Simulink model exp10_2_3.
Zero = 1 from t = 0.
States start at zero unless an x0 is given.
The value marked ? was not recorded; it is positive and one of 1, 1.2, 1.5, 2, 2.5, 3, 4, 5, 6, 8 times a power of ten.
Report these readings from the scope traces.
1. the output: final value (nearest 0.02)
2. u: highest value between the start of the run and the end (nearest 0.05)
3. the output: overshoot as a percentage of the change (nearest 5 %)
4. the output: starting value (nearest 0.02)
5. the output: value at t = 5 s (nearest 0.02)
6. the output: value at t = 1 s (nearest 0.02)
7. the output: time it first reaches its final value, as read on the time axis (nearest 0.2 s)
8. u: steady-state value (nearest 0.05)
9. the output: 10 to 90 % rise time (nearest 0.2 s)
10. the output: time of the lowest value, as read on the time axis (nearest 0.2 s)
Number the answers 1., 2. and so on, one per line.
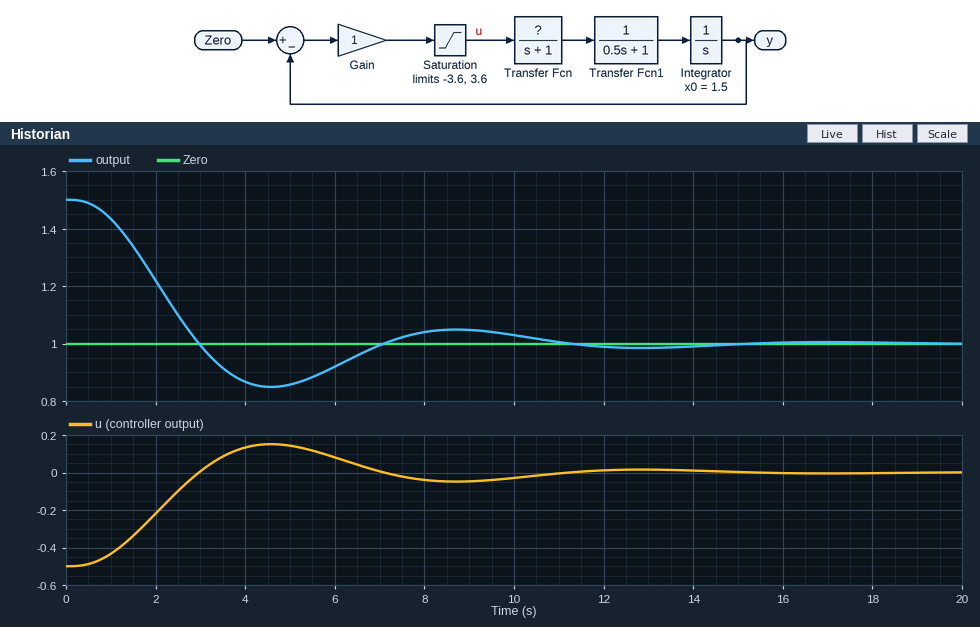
1. 1.00
2. 0.15
3. 30 %
4. 1.50
5. 0.86
6. 1.44
7. 3.0 s
8. 0.00
9. 1.8 s
10. 4.6 s
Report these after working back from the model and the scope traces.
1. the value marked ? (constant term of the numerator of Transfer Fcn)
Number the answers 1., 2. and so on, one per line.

1. 0.8
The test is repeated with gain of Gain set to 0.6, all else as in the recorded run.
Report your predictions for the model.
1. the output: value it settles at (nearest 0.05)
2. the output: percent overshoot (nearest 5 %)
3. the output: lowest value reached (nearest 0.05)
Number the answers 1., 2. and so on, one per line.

1. 1.00
2. 15 %
3. 0.95
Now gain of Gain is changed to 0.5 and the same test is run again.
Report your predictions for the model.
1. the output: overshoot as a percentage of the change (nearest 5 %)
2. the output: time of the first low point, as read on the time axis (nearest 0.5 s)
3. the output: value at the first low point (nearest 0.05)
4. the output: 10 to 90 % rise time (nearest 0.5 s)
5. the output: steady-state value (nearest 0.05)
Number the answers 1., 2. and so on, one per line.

1. 10 %
2. 7.0 s
3. 0.95
4. 3.5 s
5. 1.00
